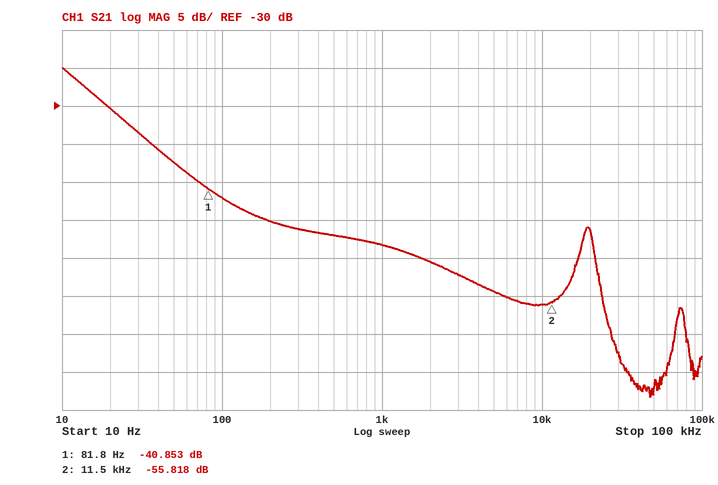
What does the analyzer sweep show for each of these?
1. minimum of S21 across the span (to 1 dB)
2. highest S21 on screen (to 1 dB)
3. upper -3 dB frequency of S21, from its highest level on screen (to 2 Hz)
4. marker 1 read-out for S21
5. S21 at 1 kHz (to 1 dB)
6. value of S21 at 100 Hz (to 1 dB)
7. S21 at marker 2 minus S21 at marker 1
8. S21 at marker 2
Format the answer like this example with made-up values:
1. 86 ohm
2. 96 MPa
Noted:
1. -68 dB
2. -25 dB
3. 14 Hz
4. -40.853 dB
5. -48 dB
6. -42 dB
7. -14.965 dB
8. -55.818 dB
